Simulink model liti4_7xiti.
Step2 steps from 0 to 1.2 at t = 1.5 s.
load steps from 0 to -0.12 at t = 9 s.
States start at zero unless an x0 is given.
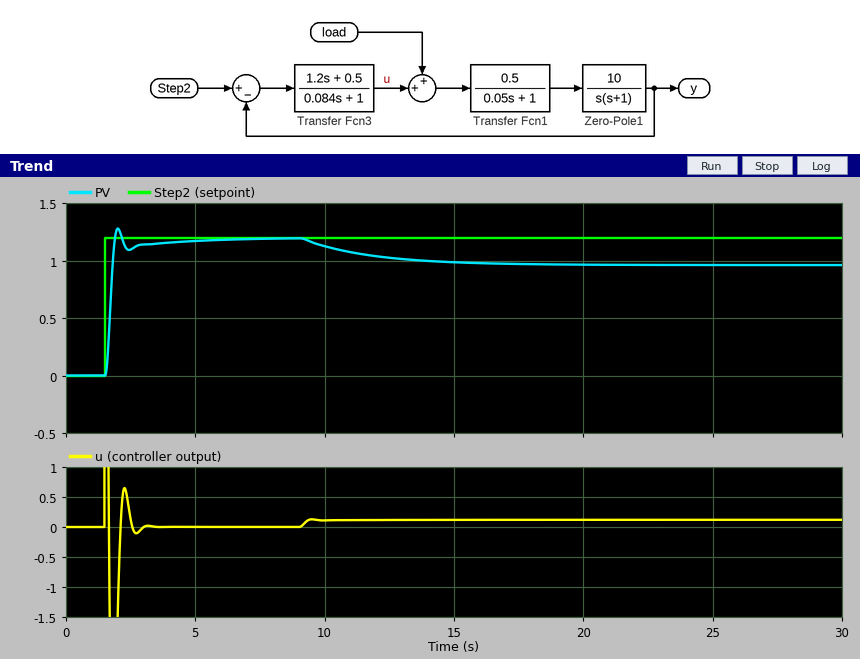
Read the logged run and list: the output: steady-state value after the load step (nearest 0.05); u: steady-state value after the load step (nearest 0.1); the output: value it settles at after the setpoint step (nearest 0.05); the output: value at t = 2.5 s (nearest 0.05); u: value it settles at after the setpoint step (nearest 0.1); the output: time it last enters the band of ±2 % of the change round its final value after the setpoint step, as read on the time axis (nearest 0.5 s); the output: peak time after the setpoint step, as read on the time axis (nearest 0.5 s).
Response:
0.95
0.1
1.20
1.10
0.0
5.5 s
2.0 s
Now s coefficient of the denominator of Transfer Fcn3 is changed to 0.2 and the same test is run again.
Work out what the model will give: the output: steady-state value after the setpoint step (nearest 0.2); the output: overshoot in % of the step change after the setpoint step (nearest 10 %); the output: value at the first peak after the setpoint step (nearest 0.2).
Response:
1.2
20 %
1.4
